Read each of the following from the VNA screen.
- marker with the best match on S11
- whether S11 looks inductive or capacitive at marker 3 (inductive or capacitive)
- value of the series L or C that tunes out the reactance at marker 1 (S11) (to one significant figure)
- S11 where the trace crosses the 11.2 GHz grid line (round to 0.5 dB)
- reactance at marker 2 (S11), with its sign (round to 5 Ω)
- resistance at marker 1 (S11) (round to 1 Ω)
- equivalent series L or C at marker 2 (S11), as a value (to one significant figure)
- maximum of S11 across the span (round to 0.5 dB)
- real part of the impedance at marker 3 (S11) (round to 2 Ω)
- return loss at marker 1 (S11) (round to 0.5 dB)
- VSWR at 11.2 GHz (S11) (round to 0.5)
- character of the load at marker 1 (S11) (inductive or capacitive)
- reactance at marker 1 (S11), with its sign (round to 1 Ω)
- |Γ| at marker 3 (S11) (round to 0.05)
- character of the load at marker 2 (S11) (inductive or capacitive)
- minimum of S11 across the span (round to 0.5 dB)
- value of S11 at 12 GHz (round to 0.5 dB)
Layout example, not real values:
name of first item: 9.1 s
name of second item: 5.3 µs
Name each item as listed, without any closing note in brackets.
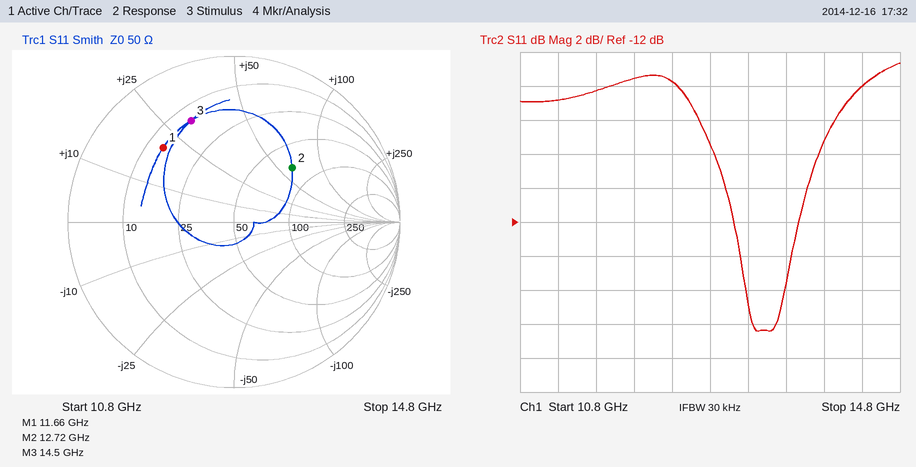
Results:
marker with the best match on S11: marker 2
whether S11 looks inductive or capacitive at marker 3: inductive
value of the series L or C that tunes out the reactance at marker 1 (S11): 700 fF
S11 where the trace crosses the 11.2 GHz grid line: -5.0 dB
reactance at marker 2 (S11), with its sign: +60 Ω
resistance at marker 1 (S11): 14 Ω
equivalent series L or C at marker 2 (S11), as a value: 800 pH
maximum of S11 across the span: -2.5 dB
real part of the impedance at marker 3 (S11): 14 Ω
return loss at marker 1 (S11): 4.0 dB
VSWR at 11.2 GHz (S11): 3.5
character of the load at marker 1 (S11): inductive
reactance at marker 1 (S11), with its sign: +20 Ω
|Γ| at marker 3 (S11): 0.65
character of the load at marker 2 (S11): inductive
minimum of S11 across the span: -18.5 dB
value of S11 at 12 GHz: -3.5 dB
